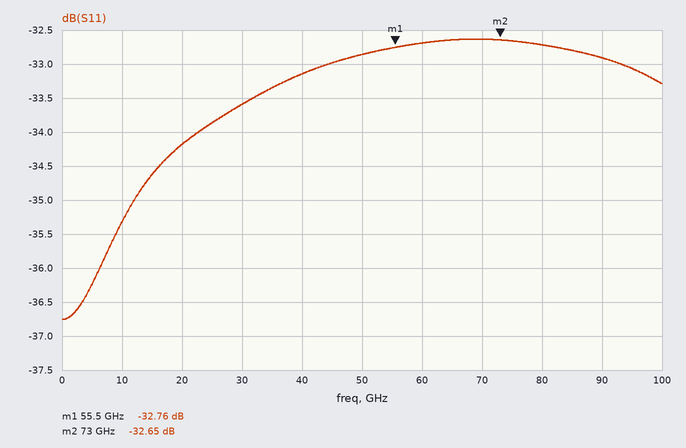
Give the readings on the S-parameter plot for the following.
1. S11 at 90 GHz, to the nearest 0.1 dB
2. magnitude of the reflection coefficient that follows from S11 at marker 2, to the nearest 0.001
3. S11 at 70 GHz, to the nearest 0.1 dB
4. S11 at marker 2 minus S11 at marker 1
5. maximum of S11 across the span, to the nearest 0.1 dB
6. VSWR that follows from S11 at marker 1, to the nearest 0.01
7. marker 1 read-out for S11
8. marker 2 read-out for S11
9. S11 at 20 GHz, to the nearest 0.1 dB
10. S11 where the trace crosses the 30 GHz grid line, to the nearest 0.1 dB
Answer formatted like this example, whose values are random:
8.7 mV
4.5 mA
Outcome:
-32.9 dB
0.023
-32.6 dB
0.11 dB
-32.6 dB
1.05
-32.76 dB
-32.65 dB
-34.2 dB
-33.6 dB
